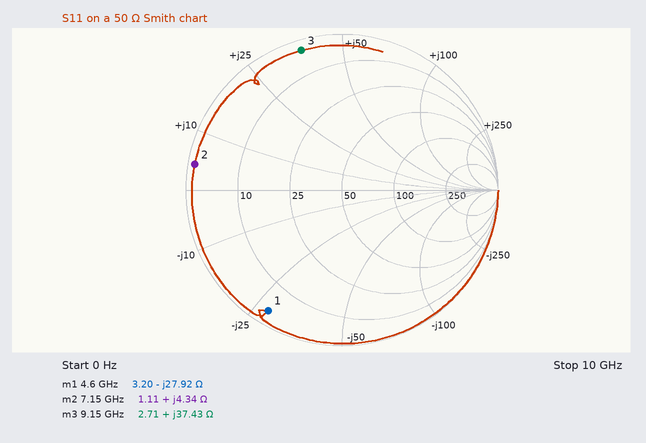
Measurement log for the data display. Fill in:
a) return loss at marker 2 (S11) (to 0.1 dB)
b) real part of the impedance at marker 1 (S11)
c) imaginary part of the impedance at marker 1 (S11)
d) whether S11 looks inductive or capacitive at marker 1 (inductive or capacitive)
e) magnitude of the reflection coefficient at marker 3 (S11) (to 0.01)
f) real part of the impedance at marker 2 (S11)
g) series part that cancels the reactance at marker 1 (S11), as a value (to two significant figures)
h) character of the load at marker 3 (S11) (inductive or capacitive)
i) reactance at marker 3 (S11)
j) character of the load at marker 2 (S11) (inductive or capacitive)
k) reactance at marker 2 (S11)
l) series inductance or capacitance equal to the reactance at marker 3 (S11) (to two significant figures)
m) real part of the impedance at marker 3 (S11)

0.4 dB
3.20 Ω
-27.92 Ω
capacitive
0.93
1.11 Ω
970 pH
inductive
+37.43 Ω
inductive
+4.34 Ω
650 pH
2.71 Ω
